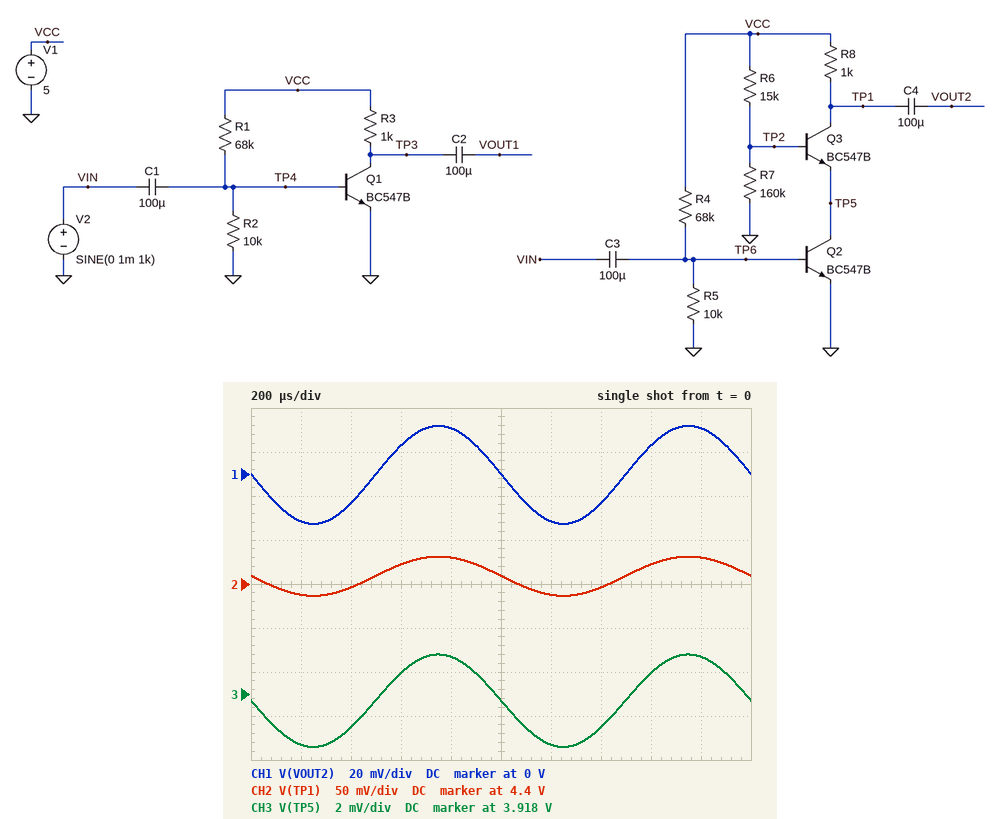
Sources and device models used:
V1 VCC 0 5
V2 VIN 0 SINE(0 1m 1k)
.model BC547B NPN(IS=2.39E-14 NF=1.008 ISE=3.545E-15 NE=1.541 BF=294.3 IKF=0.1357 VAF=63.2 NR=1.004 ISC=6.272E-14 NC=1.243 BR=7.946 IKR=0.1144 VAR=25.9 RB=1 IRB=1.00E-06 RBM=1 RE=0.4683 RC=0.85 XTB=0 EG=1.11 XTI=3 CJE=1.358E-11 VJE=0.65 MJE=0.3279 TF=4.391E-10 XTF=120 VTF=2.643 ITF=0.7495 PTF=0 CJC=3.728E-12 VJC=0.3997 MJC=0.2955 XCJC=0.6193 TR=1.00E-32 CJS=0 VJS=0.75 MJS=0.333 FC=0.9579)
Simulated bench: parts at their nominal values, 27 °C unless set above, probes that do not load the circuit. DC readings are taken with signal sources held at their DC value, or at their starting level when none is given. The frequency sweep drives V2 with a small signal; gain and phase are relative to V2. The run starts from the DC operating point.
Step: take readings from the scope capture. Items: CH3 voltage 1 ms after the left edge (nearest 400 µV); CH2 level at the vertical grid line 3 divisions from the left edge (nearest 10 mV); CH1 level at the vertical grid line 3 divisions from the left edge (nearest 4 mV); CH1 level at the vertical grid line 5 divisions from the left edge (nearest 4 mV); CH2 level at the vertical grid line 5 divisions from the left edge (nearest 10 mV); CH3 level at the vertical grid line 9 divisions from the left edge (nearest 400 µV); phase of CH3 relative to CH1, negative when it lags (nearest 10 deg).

3.9176 V
4.42 V
12 mV
0 V
4.41 V
3.9196 V
0 deg
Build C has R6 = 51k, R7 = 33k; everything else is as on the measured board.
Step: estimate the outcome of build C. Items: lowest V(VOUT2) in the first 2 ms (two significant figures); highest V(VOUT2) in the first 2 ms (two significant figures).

-22 mV
21 mV
